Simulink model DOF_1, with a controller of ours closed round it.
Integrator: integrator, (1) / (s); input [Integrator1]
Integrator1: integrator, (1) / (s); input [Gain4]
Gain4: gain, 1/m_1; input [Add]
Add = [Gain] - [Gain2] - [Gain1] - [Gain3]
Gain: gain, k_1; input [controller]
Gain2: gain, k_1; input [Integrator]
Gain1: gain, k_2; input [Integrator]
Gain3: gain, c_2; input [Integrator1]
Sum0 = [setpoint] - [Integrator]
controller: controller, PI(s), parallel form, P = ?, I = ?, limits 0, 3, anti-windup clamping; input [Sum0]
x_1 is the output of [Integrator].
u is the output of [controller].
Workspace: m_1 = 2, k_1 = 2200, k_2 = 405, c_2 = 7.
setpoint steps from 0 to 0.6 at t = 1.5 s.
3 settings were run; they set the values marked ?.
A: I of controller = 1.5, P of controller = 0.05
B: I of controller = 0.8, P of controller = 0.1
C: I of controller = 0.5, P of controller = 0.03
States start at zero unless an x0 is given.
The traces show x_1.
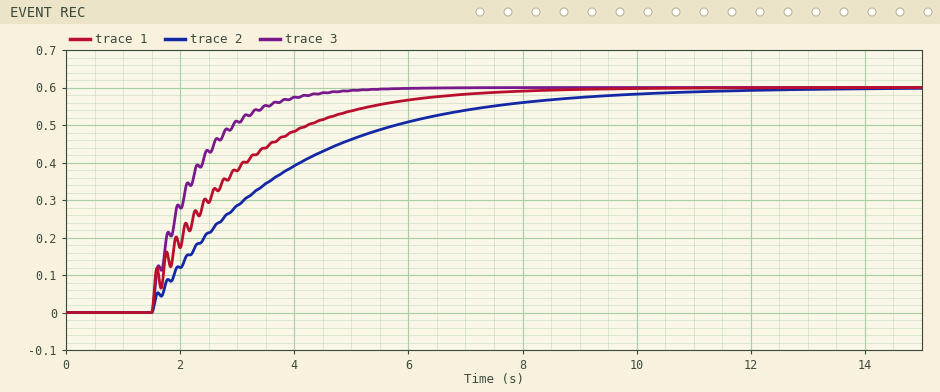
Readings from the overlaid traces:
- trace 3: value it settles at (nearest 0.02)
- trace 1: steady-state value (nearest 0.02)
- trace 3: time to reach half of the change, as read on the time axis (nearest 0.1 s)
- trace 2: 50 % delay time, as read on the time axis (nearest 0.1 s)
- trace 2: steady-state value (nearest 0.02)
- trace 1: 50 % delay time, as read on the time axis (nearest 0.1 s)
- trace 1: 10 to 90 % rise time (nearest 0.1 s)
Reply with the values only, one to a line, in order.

0.60
0.60
2.1 s
3.1 s
0.60
2.4 s
3.5 s
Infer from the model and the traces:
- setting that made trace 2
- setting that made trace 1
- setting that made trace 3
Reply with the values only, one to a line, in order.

C
B
A
